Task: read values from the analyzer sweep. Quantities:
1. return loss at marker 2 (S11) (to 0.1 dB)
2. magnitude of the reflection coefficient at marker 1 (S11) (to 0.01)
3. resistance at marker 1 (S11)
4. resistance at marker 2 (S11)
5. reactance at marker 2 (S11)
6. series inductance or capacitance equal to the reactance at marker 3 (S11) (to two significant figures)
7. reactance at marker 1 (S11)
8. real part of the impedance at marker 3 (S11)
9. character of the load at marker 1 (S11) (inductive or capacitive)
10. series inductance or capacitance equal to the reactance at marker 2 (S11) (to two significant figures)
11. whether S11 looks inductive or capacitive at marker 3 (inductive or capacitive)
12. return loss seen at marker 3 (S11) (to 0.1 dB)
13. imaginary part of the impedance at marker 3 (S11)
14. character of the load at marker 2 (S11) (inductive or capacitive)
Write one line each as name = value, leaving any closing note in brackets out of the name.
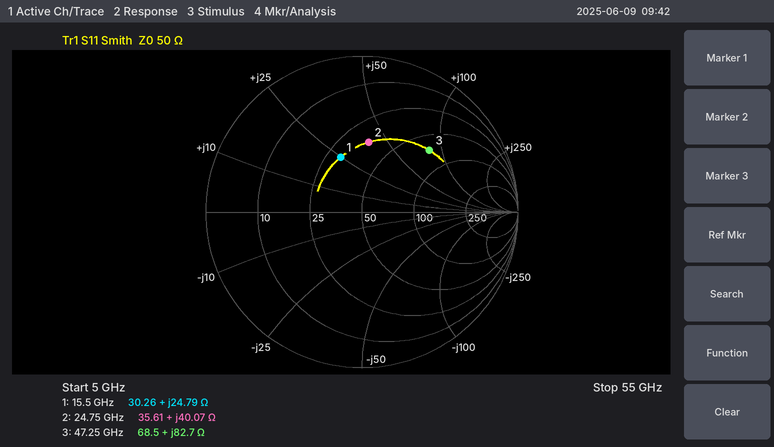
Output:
return loss at marker 2 (S11) = 6.9 dB
magnitude of the reflection coefficient at marker 1 (S11) = 0.38
resistance at marker 1 = 30.26 Ω
resistance at marker 2 = 35.61 Ω
reactance at marker 2 = +40.07 Ω
series inductance or capacitance equal to the reactance at marker 3 (S11) = 280 pH
reactance at marker 1 = +24.79 Ω
real part of the impedance at marker 3 = 68.5 Ω
character of the load at marker 1 (S11) = inductive
series inductance or capacitance equal to the reactance at marker 2 (S11) = 260 pH
whether S11 looks inductive or capacitive at marker 3 = inductive
return loss seen at marker 3 (S11) = 4.6 dB
imaginary part of the impedance at marker 3 = +82.7 Ω
character of the load at marker 2 (S11) = inductive
